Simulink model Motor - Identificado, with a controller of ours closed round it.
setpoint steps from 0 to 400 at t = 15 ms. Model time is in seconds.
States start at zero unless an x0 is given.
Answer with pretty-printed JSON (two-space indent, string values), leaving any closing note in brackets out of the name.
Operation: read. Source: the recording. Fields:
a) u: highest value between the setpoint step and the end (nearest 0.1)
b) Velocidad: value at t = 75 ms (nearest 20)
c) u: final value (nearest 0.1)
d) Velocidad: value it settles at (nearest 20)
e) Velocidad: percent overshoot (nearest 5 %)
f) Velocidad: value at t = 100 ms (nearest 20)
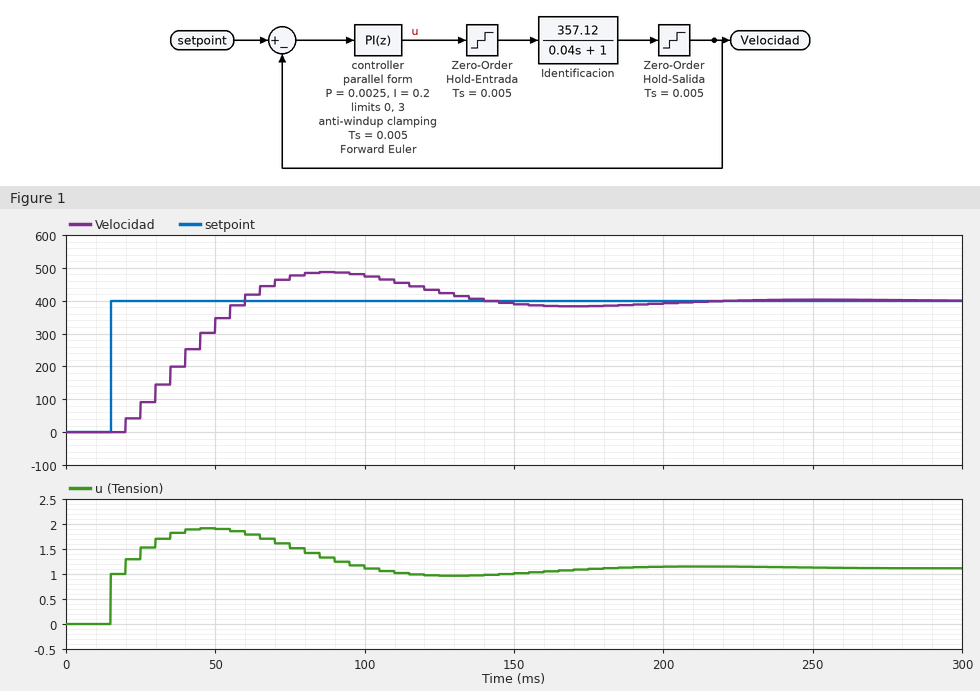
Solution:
{
  "u: highest value between the setpoint step and the end": "1.9",
  "Velocidad: value at t = 75 ms": "480",
  "u: final value": "1.1",
  "Velocidad: value it settles at": "400",
  "Velocidad: percent overshoot": "20 %",
  "Velocidad: value at t = 100 ms": "480"
}
